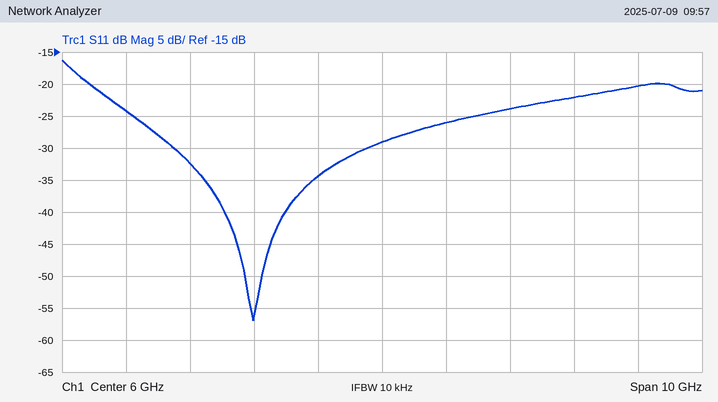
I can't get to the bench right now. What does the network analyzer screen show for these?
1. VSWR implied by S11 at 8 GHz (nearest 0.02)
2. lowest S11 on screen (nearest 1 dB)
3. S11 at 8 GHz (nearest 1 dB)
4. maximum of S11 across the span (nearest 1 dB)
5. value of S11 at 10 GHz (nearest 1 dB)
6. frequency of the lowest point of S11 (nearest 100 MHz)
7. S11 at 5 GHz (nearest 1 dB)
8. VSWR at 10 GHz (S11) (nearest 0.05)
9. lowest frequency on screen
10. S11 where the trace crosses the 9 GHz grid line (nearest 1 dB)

1.14
-57 dB
-24 dB
-16 dB
-20 dB
4.0 GHz
-34 dB
1.20
1 GHz
-22 dB
